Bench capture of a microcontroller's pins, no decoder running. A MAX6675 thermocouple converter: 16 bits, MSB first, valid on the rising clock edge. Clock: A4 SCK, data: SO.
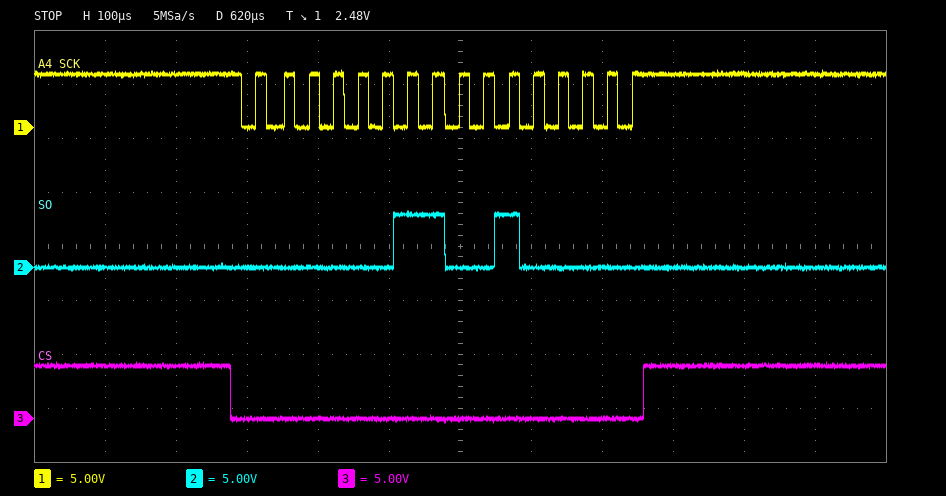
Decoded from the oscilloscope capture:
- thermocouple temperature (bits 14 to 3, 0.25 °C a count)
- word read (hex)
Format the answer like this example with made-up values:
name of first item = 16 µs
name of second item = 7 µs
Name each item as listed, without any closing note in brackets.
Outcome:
thermocouple temperature = 25.00 °C
word read = 0x0320
